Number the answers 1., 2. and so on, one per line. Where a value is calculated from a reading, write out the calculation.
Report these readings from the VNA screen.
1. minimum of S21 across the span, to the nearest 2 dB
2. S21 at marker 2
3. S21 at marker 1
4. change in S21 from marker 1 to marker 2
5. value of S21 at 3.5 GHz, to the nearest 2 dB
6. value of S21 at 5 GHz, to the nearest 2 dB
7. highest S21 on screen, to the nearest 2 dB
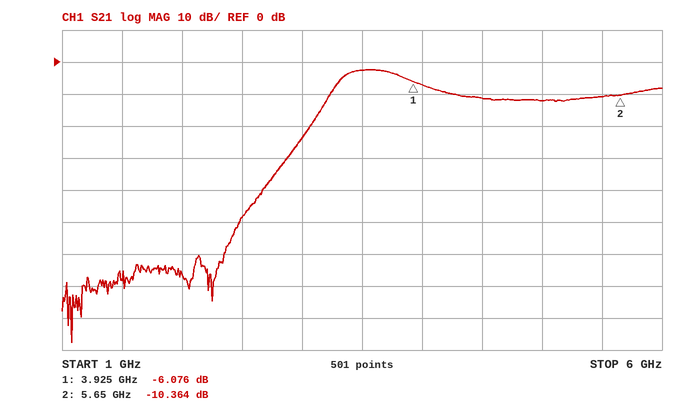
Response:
1. -88 dB
2. -10.364 dB
3. -6.076 dB
4. -10.364 − (-6.076) = -4.288 dB
5. -2 dB
6. -12 dB
7. -2 dB
